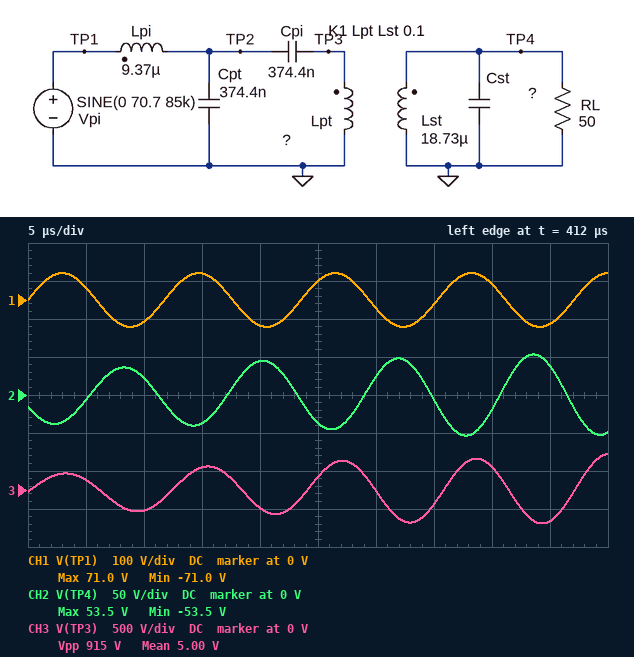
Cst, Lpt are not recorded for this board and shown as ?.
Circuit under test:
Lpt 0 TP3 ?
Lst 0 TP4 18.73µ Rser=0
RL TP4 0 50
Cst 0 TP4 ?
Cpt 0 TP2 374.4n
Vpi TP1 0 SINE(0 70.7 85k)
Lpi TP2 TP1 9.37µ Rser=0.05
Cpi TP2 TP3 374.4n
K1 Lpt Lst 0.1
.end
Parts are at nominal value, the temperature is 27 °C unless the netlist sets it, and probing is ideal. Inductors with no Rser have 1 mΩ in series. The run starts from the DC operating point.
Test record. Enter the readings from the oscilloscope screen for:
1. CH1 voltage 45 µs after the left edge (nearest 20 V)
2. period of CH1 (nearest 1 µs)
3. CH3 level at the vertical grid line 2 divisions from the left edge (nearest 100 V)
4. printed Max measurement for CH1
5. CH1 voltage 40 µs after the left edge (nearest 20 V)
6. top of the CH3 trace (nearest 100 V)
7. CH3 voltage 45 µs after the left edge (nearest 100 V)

-60 V
12 µs
-300 V
71.0 V
40 V
500 V
-400 V
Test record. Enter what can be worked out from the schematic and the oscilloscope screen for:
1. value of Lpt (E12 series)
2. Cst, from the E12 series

47 µH
270 nF
